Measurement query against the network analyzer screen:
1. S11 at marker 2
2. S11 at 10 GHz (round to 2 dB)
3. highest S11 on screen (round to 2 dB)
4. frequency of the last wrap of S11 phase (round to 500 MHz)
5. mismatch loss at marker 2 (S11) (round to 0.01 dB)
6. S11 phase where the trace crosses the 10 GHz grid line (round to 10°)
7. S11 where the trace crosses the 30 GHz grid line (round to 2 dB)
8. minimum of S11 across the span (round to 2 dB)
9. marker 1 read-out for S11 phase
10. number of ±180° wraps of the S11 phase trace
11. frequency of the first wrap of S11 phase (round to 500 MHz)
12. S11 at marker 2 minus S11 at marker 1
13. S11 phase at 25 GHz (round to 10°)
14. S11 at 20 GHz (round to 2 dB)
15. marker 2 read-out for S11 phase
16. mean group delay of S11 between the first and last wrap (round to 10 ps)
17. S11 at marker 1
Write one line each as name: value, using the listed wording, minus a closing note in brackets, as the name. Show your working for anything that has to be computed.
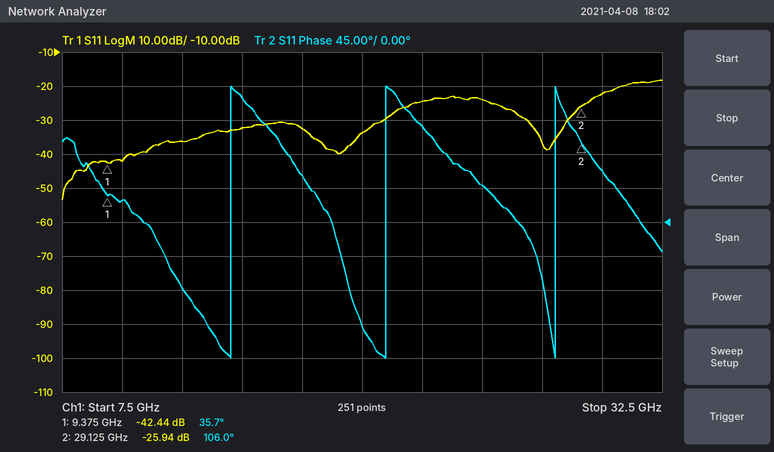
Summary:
S11 at marker 2: -25.94 dB
S11 at 10 GHz: -42 dB
highest S11 on screen: -18 dB
frequency of the last wrap of S11 phase: 28.0 GHz
mismatch loss at marker 2 (S11): −10 log10(1 − 10^(-25.94/10)) ≈ 0.01 dB
S11 phase where the trace crosses the 10 GHz grid line: 30°
S11 where the trace crosses the 30 GHz grid line: -22 dB
minimum of S11 across the span: -54 dB
marker 1 read-out for S11 phase: 35.7°
number of ±180° wraps of the S11 phase trace: 3
frequency of the first wrap of S11 phase: 14.5 GHz
S11 at marker 2 minus S11 at marker 1: -25.94 − (-42.44) = 16.50 dB
S11 phase at 25 GHz: 50°
S11 at 20 GHz: -34 dB
marker 2 read-out for S11 phase: 106.0°
mean group delay of S11 between the first and last wrap: 2 cycles / (28.0 GHz − 14.5 GHz) ≈ 148 ps, so 150 ps to the nearest 10 ps
S11 at marker 1: -42.44 dB
